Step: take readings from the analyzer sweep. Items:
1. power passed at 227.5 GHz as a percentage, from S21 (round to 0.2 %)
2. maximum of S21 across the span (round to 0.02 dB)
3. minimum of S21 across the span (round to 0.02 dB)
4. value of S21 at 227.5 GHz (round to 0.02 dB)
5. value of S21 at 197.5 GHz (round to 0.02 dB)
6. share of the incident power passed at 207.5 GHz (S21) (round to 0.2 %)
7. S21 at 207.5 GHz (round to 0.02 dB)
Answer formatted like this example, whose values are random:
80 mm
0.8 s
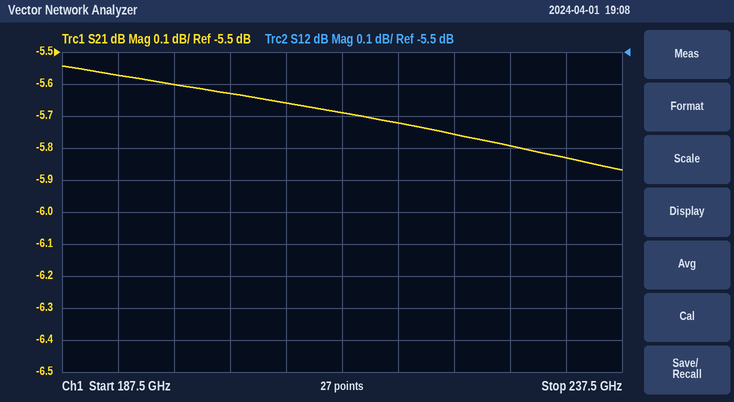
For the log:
26.4 %
-5.54 dB
-5.86 dB
-5.80 dB
-5.60 dB
27.2 %
-5.66 dB
